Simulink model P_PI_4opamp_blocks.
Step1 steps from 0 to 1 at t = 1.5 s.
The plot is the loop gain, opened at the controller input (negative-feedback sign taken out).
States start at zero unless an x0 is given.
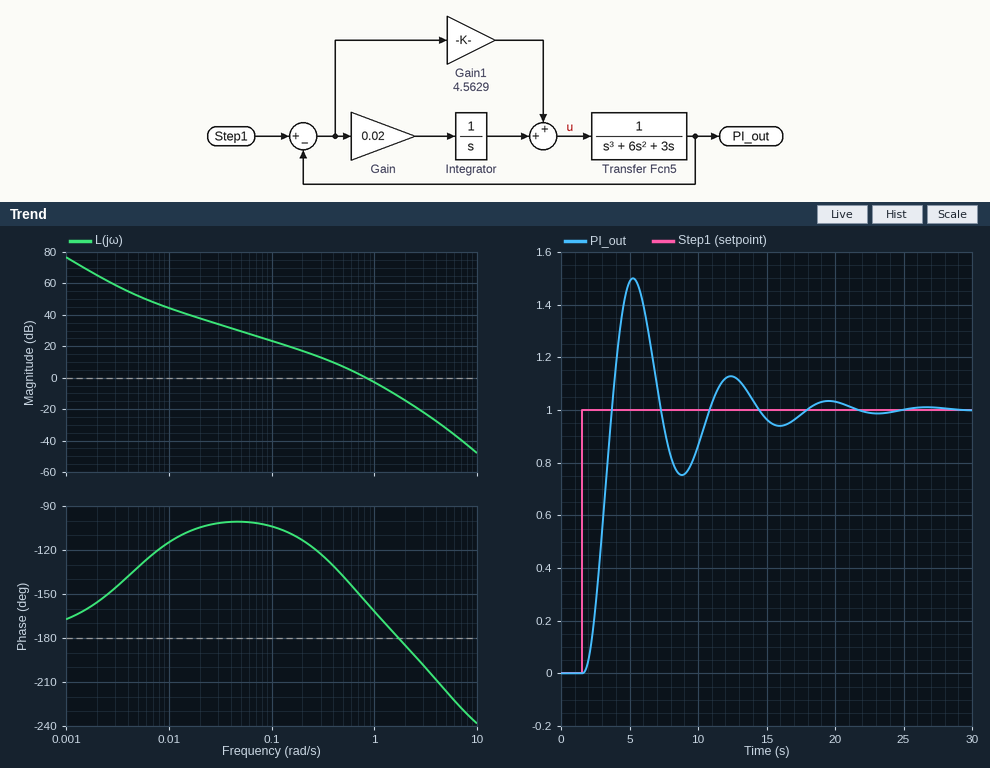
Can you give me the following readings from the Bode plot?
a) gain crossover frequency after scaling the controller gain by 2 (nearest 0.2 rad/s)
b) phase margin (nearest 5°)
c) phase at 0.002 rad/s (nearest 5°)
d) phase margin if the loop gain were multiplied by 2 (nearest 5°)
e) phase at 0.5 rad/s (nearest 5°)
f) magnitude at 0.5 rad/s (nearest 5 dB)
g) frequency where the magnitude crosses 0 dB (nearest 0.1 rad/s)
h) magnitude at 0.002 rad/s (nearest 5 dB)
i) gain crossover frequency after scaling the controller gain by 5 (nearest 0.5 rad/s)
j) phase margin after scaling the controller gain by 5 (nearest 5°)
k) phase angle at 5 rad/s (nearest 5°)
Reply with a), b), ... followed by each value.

a) 1.2 rad/s
b) 25°
c) -155°
d) 10°
e) -140°
f) 5 dB
g) 0.8 rad/s
h) 65 dB
i) 2.0 rad/s
j) -5°
k) -215°
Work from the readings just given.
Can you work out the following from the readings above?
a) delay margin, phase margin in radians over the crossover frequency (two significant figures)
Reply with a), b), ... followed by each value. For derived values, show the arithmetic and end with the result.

a) 25 × π / 180 / 0.8 = 0.55 s
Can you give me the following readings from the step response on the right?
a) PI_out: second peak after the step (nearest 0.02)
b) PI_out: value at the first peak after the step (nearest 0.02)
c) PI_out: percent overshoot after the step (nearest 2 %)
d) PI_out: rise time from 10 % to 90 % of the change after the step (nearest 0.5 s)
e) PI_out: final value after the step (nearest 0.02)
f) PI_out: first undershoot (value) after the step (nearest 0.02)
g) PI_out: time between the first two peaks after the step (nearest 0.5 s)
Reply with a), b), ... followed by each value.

a) 1.12
b) 1.50
c) 50 %
d) 1.5 s
e) 1.00
f) 0.76
g) 7.0 s
